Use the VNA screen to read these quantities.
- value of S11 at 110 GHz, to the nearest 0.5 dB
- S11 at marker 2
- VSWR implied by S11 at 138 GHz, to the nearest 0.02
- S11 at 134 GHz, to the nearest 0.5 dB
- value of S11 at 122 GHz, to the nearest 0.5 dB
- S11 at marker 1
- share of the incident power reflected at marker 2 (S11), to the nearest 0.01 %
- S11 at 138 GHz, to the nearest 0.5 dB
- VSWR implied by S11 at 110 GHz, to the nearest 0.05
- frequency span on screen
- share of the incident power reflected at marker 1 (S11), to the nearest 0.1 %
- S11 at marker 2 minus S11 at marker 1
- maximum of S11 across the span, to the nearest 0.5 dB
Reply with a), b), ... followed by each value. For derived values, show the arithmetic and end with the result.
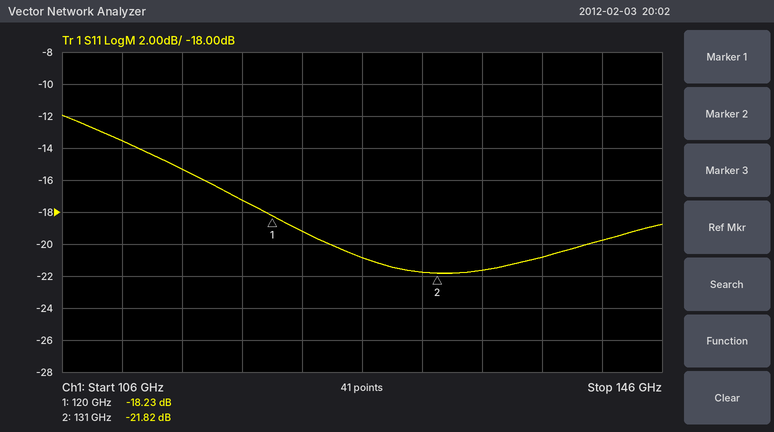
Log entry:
a) -13.5 dB
b) -21.82 dB
c) |Γ| = 10^(-21/20) = 0.0891; VSWR = (1 + 0.0891)/(1 − 0.0891) ≈ 1.20
d) -21.5 dB
e) -19.0 dB
f) -18.23 dB
g) 10^(-21.82/10) ≈ 0.66 %
h) -21.0 dB
i) |Γ| = 10^(-13.5/20) = 0.2113; VSWR = (1 + 0.2113)/(1 − 0.2113) ≈ 1.54, so 1.55 to the nearest 0.05
j) 40 GHz
k) 10^(-18.23/10) ≈ 1.5 %
l) -21.82 − (-18.23) = -3.59 dB
m) -12.0 dB
